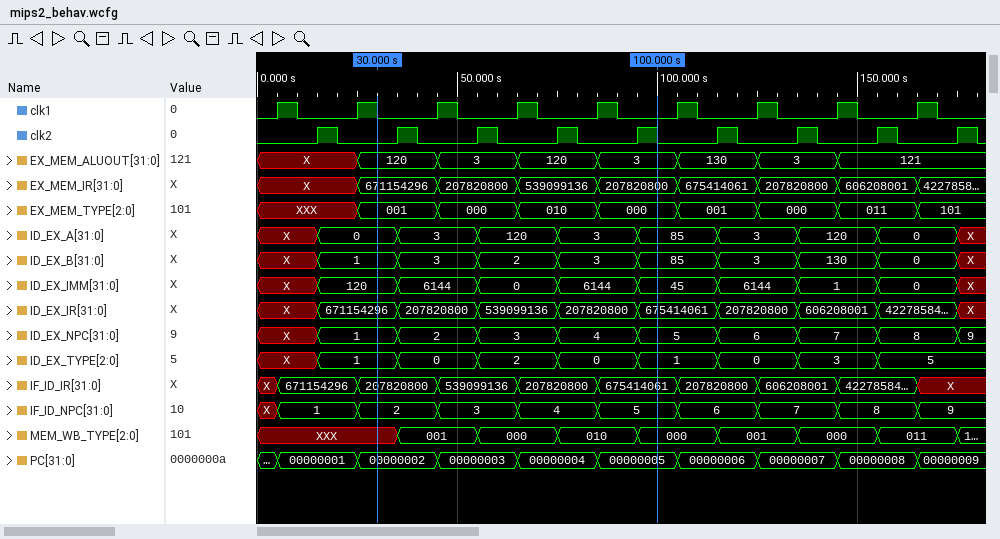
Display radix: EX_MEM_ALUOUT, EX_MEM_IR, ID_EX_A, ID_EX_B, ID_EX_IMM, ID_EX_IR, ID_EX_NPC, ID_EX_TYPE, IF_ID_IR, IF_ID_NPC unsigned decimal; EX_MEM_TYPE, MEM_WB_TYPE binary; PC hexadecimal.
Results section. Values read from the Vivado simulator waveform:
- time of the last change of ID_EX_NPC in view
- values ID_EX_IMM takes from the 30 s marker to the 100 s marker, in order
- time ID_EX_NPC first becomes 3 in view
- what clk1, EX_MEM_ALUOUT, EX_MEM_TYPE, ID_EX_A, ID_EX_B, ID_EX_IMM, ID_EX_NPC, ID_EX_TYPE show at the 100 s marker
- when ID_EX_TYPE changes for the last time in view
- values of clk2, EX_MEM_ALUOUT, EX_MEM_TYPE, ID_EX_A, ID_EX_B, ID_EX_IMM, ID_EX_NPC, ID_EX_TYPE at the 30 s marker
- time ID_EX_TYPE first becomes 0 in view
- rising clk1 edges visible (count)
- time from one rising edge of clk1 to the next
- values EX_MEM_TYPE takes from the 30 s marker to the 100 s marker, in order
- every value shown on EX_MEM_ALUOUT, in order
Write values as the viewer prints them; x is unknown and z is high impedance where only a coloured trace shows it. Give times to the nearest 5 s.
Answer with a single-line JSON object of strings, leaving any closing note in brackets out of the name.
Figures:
{"time of the last change of ID_EX_NPC in view": "175 s", "values ID_EX_IMM takes from the 30 s marker to the 100 s marker, in order": "120, 6144, 0, 6144, 45", "time ID_EX_NPC first becomes 3 in view": "55 s", "what clk1, EX_MEM_ALUOUT, EX_MEM_TYPE, ID_EX_A, ID_EX_B, ID_EX_IMM, ID_EX_NPC, ID_EX_TYPE show at the 100 s marker": "clk1=0, EX_MEM_ALUOUT=3, EX_MEM_TYPE=000, ID_EX_A=85, ID_EX_B=85, ID_EX_IMM=45, ID_EX_NPC=5, ID_EX_TYPE=1", "when ID_EX_TYPE changes for the last time in view": "155 s", "values of clk2, EX_MEM_ALUOUT, EX_MEM_TYPE, ID_EX_A, ID_EX_B, ID_EX_IMM, ID_EX_NPC, ID_EX_TYPE at the 30 s marker": "clk2=0, EX_MEM_ALUOUT=120, EX_MEM_TYPE=001, ID_EX_A=0, ID_EX_B=1, ID_EX_IMM=120, ID_EX_NPC=1, ID_EX_TYPE=1", "time ID_EX_TYPE first becomes 0 in view": "35 s", "rising clk1 edges visible": "9", "time from one rising edge of clk1 to the next": "20 s", "values EX_MEM_TYPE takes from the 30 s marker to the 100 s marker, in order": "001, 000, 010, 000", "every value shown on EX_MEM_ALUOUT, in order": "X, 120, 3, 120, 3, 130, 3, 121"}
